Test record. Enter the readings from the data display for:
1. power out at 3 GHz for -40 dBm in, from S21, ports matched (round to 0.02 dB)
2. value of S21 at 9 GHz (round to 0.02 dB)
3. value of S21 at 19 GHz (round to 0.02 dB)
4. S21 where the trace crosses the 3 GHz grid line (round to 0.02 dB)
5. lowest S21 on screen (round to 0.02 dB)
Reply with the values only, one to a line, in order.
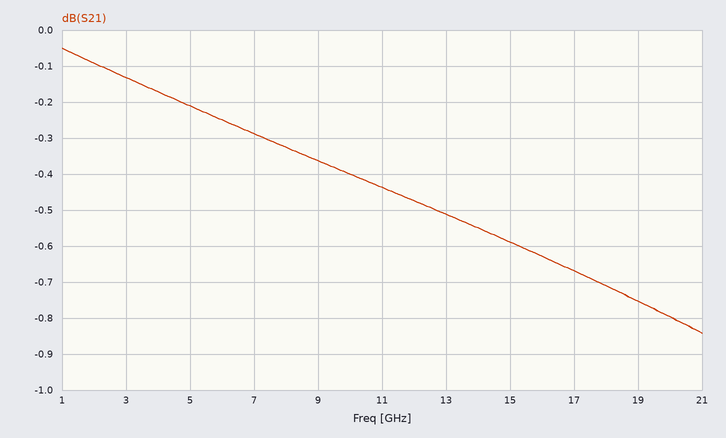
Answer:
-40.14 dBm
-0.36 dB
-0.76 dB
-0.14 dB
-0.84 dB
